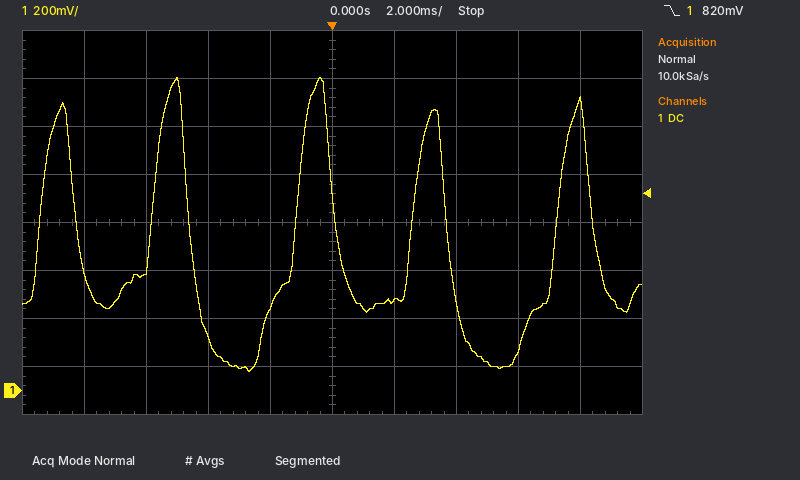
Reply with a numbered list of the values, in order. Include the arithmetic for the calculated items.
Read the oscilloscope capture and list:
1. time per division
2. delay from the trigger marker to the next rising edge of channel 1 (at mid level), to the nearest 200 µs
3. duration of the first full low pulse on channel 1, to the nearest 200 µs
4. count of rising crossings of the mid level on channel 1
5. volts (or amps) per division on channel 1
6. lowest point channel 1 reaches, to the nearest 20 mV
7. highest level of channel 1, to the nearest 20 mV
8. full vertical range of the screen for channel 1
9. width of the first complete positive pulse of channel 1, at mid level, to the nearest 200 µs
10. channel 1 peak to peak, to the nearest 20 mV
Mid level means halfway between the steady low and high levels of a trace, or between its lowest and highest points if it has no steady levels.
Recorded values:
1. 2 ms
2. 2.6 ms
3. 2.4 ms
4. 5
5. 200 mV
6. 80 mV
7. 1.30 V
8. 1.6 V
9. 1.2 ms
10. 1.30 V − (80 mV) = 1.22 V
